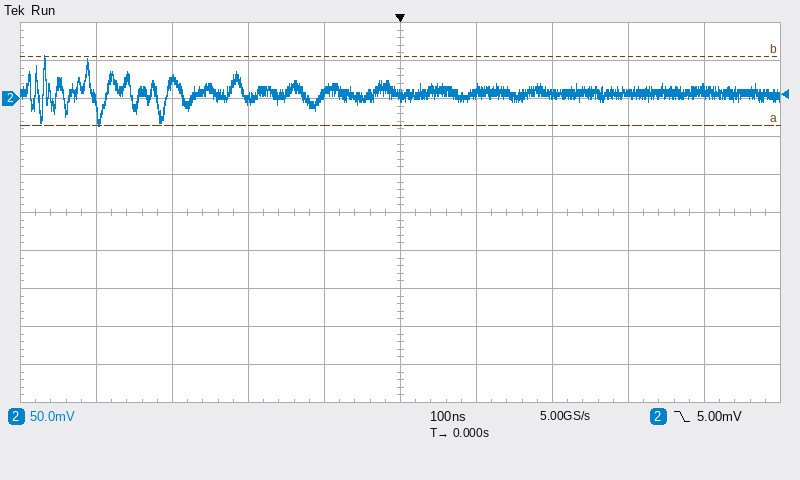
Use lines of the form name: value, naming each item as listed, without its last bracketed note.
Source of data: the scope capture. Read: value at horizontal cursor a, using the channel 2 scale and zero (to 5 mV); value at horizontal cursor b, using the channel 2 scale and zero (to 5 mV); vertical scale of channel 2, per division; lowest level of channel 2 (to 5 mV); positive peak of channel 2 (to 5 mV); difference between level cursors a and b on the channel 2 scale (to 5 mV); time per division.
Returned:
value at horizontal cursor a, using the channel 2 scale and zero: -35 mV
value at horizontal cursor b, using the channel 2 scale and zero: 55 mV
vertical scale of channel 2, per division: 50 mV
lowest level of channel 2: -35 mV
positive peak of channel 2: 55 mV
difference between level cursors a and b on the channel 2 scale: 90 mV
time per division: 100 ns
